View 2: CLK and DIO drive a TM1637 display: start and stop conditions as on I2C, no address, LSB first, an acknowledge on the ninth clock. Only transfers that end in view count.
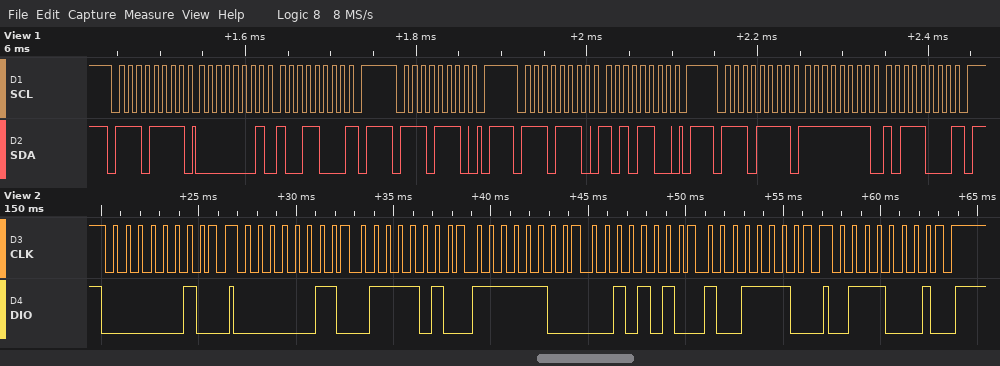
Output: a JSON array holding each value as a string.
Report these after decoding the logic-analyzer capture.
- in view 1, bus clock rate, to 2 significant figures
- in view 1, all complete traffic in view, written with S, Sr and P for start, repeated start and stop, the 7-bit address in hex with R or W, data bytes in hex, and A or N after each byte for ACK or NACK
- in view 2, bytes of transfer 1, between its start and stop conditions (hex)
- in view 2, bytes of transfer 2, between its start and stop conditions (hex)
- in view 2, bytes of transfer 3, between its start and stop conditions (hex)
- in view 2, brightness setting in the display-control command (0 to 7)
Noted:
["100 kHz", "S 77R A 01 A 98 N P S 77W A P S 77W A AC A P S 77R A FF A B8 N P", "40", "C0 5E 3F 54 79", "8E", "6"]
